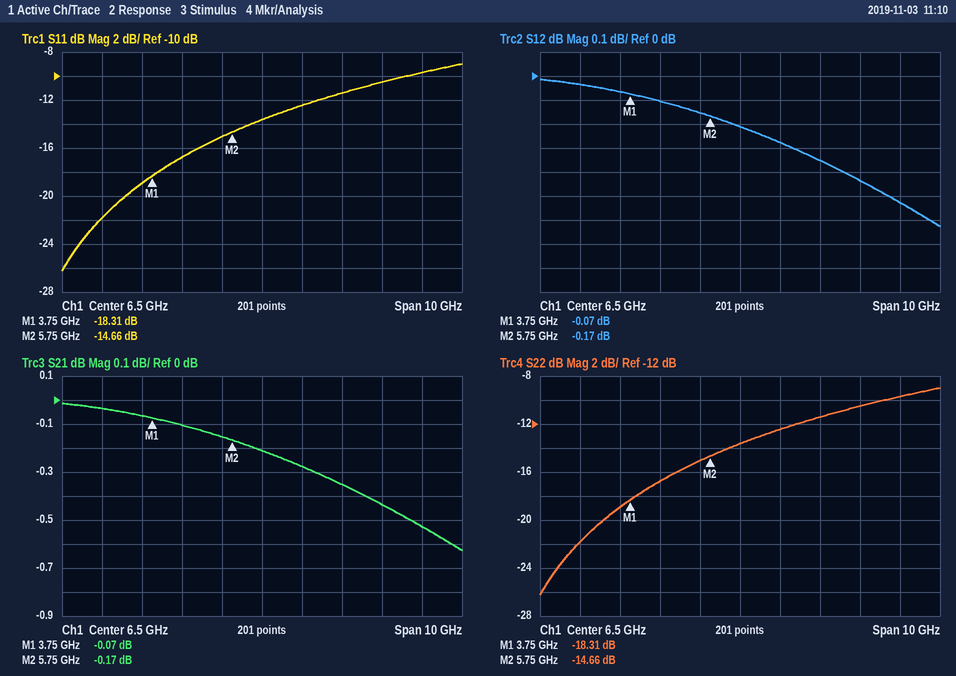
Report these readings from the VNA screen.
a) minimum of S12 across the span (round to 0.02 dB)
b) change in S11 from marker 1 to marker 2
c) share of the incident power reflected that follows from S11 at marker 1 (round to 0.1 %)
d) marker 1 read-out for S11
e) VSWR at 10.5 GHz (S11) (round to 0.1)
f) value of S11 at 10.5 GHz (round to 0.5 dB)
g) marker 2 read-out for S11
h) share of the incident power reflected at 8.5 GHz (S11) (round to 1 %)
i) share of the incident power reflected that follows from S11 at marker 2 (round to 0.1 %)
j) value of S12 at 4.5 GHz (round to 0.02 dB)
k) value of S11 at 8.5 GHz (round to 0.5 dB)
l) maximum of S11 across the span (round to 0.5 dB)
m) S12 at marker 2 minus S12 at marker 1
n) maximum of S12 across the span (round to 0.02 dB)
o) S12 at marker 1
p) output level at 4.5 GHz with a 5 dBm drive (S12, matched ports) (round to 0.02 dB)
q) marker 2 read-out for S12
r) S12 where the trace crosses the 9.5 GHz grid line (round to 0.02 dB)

-0.62 dB
3.65 dB
1.5 %
-18.31 dB
2.0
-9.5 dB
-14.66 dB
7 %
3.4 %
-0.10 dB
-11.5 dB
-9.0 dB
-0.10 dB
-0.02 dB
-0.07 dB
4.90 dBm
-0.17 dB
-0.44 dB
